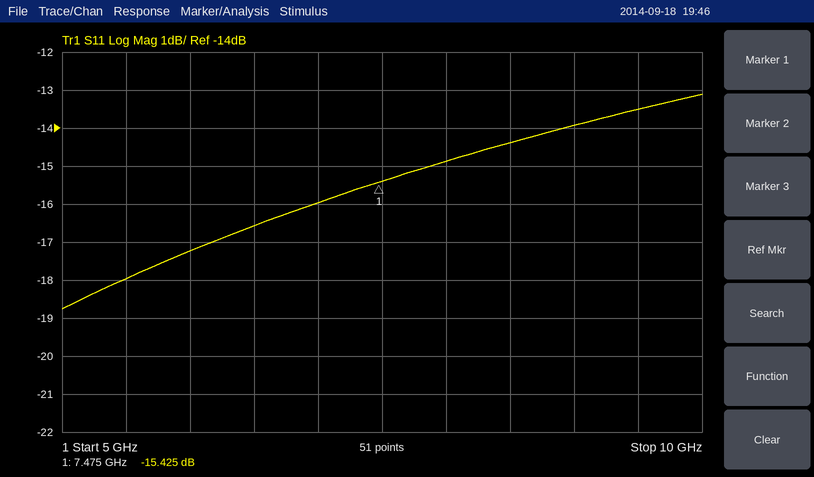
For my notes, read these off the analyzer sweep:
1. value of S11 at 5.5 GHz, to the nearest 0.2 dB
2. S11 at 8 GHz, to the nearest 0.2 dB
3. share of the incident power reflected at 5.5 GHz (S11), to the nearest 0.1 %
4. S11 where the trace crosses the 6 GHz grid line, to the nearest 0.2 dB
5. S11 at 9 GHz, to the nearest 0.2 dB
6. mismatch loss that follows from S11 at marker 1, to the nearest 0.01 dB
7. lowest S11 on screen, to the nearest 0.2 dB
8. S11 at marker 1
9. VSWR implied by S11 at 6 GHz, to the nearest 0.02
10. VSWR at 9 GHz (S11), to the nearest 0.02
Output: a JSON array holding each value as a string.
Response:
["-18.0 dB", "-14.8 dB", "1.6 %", "-17.2 dB", "-14.0 dB", "0.13 dB", "-18.8 dB", "-15.425 dB", "1.32", "1.50"]
